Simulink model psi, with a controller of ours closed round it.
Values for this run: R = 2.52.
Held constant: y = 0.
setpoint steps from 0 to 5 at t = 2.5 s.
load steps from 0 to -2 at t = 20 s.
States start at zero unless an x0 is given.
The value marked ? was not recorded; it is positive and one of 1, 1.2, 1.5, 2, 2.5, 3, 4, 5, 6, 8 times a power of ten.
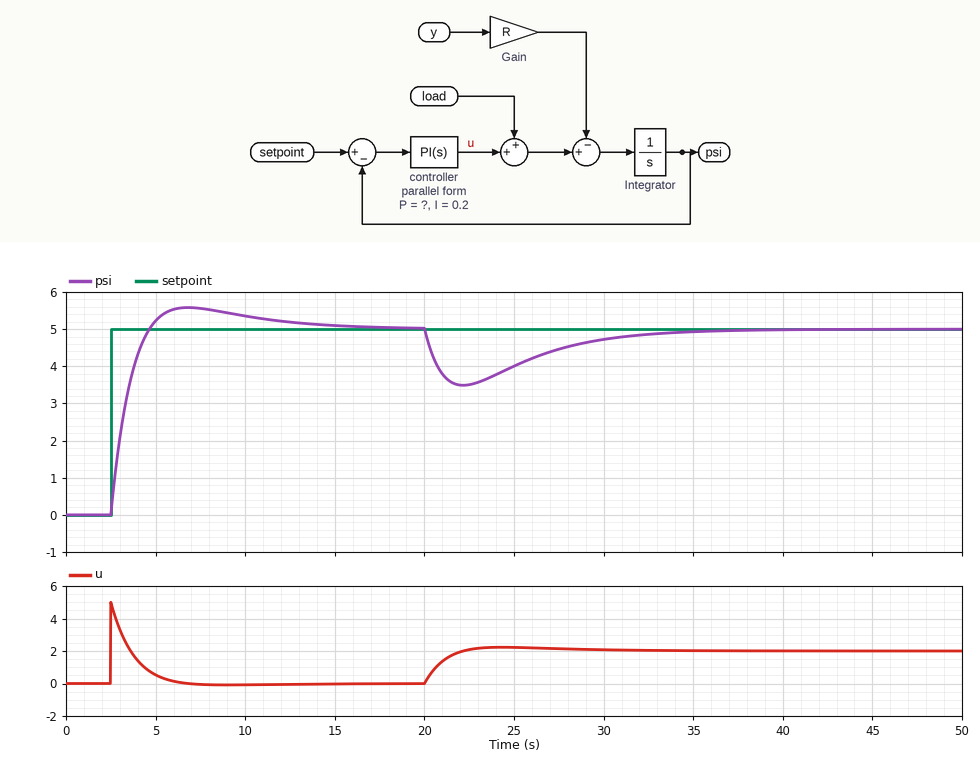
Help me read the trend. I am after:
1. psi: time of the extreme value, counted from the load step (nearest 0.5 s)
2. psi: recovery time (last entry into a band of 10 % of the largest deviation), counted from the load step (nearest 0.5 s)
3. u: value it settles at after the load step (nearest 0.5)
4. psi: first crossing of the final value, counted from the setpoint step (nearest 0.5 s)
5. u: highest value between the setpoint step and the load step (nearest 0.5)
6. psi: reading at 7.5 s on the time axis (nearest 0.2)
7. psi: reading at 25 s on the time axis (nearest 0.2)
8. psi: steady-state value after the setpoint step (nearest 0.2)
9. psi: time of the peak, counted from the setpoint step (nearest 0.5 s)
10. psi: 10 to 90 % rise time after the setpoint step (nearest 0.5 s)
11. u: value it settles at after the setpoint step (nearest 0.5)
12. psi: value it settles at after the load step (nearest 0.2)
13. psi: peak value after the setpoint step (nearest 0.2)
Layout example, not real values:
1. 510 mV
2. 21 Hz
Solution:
1. 2.0 s
2. 12.0 s
3. 2.0
4. 2.0 s
5. 5.0
6. 5.6
7. 4.0
8. 5.0
9. 4.5 s
10. 1.5 s
11. 0.0
12. 5.0
13. 5.6
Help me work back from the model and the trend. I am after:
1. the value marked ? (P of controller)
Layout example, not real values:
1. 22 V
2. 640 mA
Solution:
1. 1
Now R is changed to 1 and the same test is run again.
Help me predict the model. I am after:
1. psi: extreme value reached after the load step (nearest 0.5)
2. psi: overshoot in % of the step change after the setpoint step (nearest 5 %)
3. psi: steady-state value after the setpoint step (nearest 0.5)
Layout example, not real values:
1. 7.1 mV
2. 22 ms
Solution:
1. 3.5
2. 10 %
3. 5.0
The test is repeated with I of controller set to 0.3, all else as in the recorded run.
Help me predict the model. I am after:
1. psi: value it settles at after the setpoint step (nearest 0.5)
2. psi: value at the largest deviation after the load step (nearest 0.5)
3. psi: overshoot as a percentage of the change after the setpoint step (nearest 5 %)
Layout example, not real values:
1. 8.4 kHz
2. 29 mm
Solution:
1. 5.0
2. 3.5
3. 15 %
